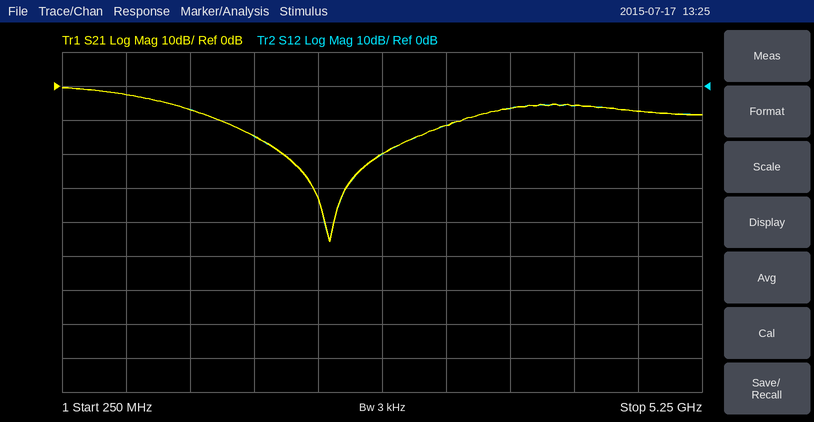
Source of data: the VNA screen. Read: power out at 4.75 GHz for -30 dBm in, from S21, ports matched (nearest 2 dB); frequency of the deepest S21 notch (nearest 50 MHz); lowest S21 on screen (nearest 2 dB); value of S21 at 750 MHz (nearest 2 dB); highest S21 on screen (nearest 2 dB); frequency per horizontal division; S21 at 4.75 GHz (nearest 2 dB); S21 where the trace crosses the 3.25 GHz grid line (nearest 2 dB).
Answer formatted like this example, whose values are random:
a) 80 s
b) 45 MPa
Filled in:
a) -38 dBm
b) 2.35 GHz
c) -46 dB
d) -2 dB
e) 0 dB
f) 500 MHz
g) -8 dB
h) -12 dB
